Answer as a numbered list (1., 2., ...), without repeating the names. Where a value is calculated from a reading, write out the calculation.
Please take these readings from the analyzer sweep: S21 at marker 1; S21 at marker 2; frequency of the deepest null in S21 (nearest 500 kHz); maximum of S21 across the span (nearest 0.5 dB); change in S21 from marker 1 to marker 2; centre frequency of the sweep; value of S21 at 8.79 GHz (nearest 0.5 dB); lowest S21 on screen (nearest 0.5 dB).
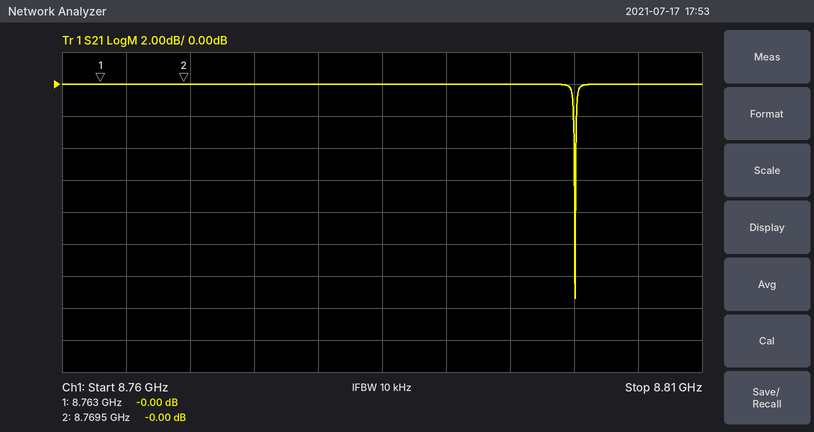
1. -0.00 dB
2. -0.00 dB
3. 8.8000 GHz
4. 0.0 dB
5. -0 − (-0) = 0.00 dB
6. 8.785 GHz
7. 0.0 dB
8. -13.5 dB
